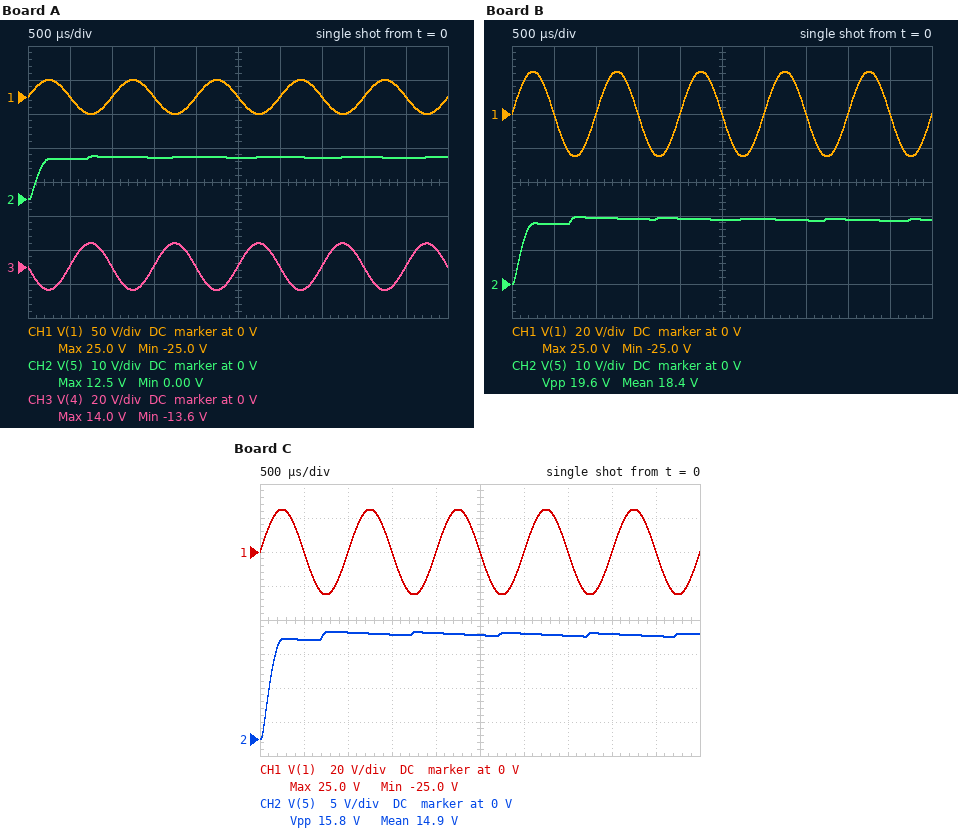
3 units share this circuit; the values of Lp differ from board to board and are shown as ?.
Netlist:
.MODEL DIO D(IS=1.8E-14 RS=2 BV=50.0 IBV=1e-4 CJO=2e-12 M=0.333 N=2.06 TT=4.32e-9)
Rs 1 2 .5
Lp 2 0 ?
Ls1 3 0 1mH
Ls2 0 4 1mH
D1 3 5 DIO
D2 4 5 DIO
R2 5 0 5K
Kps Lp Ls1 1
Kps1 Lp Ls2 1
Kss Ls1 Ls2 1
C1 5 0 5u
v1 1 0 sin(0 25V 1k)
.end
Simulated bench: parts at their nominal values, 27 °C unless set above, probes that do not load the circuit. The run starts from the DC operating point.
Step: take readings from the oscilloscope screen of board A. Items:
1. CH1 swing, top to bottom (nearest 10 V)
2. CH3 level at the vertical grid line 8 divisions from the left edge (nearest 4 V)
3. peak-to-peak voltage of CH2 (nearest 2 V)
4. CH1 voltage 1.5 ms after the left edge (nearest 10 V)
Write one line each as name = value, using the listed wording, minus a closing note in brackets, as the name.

CH1 swing, top to bottom = 50 V
CH3 level at the vertical grid line 8 divisions from the left edge = 0 V
peak-to-peak voltage of CH2 = 12 V
CH1 voltage 1.5 ms after the left edge = 0 V
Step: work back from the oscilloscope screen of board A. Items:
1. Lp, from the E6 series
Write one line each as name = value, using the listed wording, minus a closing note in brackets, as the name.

Lp, from the E6 series = 3.3 mH
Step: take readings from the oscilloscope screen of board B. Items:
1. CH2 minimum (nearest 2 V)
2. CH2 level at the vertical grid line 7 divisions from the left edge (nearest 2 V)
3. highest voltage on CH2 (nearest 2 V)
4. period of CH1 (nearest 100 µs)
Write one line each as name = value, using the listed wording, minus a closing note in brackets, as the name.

CH2 minimum = 0 V
CH2 level at the vertical grid line 7 divisions from the left edge = 18 V
highest voltage on CH2 = 20 V
period of CH1 = 1.0 ms
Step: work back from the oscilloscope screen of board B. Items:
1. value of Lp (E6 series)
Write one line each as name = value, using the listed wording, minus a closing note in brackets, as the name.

value of Lp = 1.5 mH
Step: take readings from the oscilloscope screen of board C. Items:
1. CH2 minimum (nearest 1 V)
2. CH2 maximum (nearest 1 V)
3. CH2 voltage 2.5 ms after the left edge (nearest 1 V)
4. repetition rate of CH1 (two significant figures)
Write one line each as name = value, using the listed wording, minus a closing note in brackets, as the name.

CH2 minimum = 0 V
CH2 maximum = 16 V
CH2 voltage 2.5 ms after the left edge = 15 V
repetition rate of CH1 = 1.0 kHz
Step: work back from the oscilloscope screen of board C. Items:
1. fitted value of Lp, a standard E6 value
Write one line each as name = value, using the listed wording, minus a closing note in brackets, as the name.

fitted value of Lp, a standard E6 value = 2.2 mH
